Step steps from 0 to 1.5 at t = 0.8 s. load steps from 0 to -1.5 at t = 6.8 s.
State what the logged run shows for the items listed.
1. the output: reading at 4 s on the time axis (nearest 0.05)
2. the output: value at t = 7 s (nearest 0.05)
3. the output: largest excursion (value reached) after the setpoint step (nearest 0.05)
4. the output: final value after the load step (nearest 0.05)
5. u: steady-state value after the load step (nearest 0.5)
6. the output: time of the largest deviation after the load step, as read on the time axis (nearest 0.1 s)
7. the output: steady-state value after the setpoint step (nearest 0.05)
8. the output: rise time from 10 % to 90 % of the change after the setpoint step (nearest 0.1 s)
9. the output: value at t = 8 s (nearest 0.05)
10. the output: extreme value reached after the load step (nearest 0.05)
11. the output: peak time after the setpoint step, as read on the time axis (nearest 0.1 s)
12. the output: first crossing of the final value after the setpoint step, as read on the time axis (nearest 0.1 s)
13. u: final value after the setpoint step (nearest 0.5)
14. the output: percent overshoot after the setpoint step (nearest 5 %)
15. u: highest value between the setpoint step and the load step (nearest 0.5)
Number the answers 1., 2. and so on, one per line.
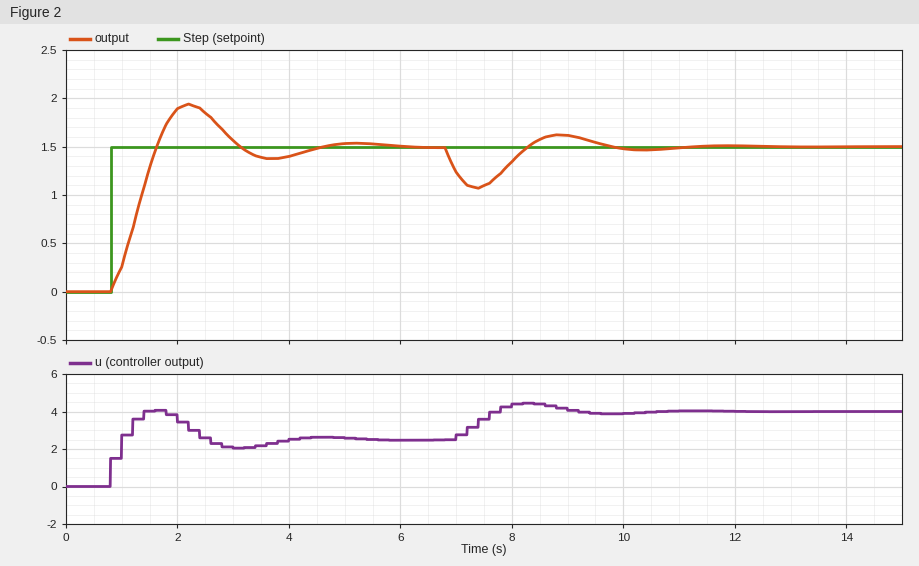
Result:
1. 1.40
2. 1.25
3. 1.95
4. 1.50
5. 4.0
6. 7.4 s
7. 1.50
8. 0.6 s
9. 1.35
10. 1.05
11. 2.2 s
12. 1.6 s
13. 2.5
14. 30 %
15. 4.0
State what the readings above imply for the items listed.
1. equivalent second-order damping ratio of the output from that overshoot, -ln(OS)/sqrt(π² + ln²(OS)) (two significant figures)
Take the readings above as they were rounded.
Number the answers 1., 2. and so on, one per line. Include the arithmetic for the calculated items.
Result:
1. ln(0.3) = -1.204; 1.204 / sqrt(9.870 + 1.450) = 0.36
